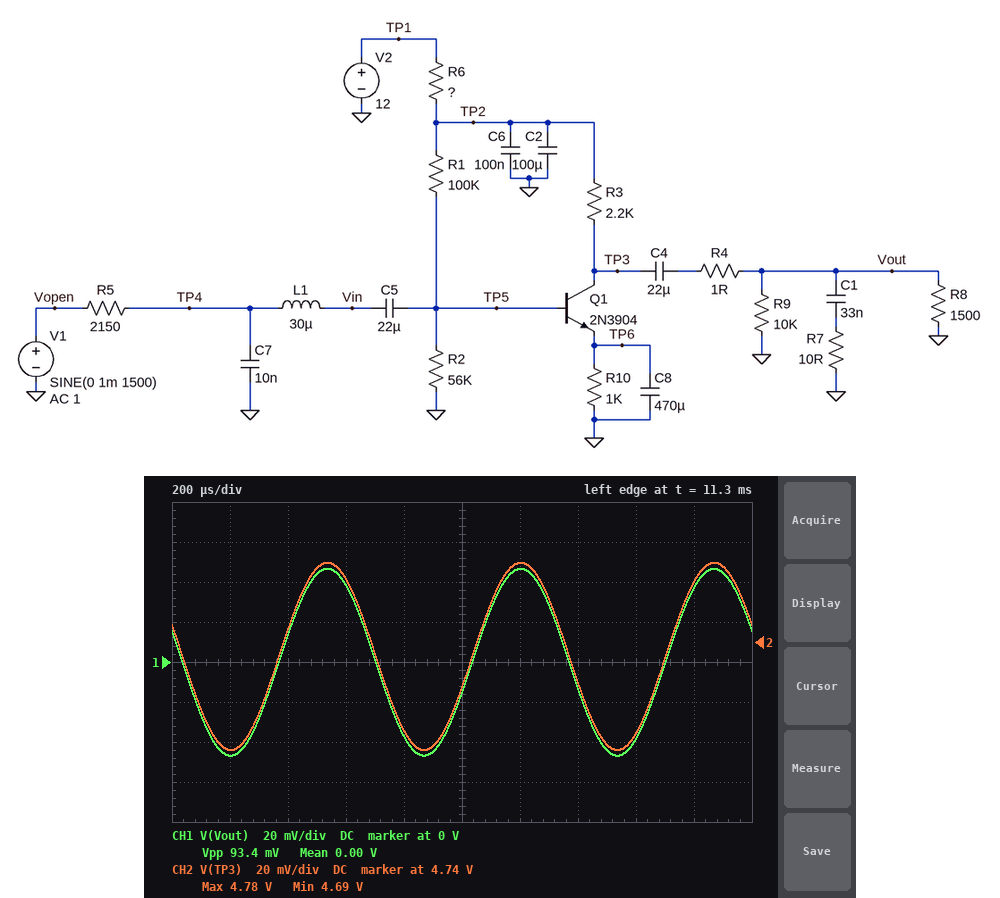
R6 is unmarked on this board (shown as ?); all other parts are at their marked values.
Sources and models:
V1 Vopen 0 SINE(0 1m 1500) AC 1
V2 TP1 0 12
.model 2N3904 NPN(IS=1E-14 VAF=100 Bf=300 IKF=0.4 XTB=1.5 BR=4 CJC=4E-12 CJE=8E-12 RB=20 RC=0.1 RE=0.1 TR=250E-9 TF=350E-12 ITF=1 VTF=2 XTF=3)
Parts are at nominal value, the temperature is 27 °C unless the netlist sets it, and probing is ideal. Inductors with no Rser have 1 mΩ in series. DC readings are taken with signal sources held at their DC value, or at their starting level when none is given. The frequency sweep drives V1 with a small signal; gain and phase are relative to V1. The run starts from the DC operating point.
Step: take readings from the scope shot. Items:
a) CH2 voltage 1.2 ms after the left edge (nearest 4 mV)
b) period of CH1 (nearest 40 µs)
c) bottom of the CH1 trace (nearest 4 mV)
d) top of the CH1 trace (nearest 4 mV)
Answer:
4.780 V
680 µs
-48 mV
48 mV
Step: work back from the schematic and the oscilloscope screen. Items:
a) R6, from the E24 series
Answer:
180 Ω
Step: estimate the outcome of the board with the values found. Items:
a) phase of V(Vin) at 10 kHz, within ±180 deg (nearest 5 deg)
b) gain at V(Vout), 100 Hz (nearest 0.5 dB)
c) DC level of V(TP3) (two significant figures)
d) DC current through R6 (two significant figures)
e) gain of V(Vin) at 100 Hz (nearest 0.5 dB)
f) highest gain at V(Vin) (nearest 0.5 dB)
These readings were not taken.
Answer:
-35 deg
33.5 dB
4.7 V
3.1 mA
-5.0 dB
0 dB
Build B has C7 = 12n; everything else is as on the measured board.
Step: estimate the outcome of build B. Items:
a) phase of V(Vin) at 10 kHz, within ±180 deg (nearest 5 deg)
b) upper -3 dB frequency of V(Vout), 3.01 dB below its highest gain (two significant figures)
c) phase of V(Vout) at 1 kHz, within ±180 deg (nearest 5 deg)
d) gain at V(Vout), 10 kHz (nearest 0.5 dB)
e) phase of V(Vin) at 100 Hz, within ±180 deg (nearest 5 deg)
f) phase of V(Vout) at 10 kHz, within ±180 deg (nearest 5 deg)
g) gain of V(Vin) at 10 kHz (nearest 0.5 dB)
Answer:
-40 deg
4.9 kHz
165 deg
25.5 dB
-10 deg
80 deg
-8.0 dB
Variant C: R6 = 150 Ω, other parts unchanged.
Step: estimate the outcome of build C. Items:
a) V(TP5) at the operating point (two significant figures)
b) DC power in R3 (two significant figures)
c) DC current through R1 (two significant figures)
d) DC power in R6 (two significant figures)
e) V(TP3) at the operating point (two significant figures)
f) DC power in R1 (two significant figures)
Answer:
3.8 V
21 mW
78 µA
1.5 mW
4.8 V
600 µW
